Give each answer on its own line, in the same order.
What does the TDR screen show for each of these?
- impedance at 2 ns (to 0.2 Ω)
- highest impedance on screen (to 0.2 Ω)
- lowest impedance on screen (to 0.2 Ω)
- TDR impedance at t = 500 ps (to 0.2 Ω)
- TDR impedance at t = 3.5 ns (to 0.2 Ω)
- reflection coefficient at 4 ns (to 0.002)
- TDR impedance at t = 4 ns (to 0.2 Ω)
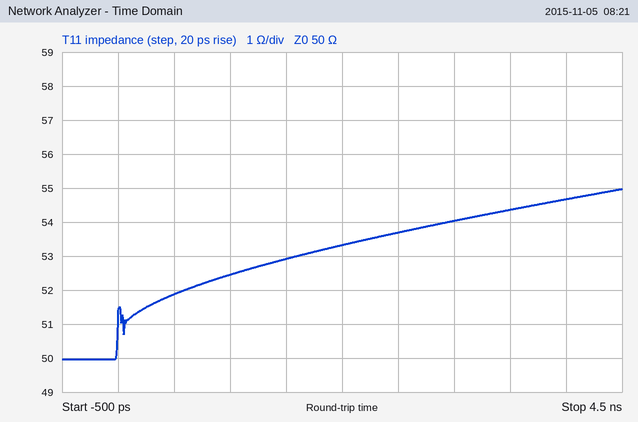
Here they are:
53.4 Ω
55.0 Ω
50.0 Ω
51.8 Ω
54.4 Ω
+0.044
54.6 Ω
